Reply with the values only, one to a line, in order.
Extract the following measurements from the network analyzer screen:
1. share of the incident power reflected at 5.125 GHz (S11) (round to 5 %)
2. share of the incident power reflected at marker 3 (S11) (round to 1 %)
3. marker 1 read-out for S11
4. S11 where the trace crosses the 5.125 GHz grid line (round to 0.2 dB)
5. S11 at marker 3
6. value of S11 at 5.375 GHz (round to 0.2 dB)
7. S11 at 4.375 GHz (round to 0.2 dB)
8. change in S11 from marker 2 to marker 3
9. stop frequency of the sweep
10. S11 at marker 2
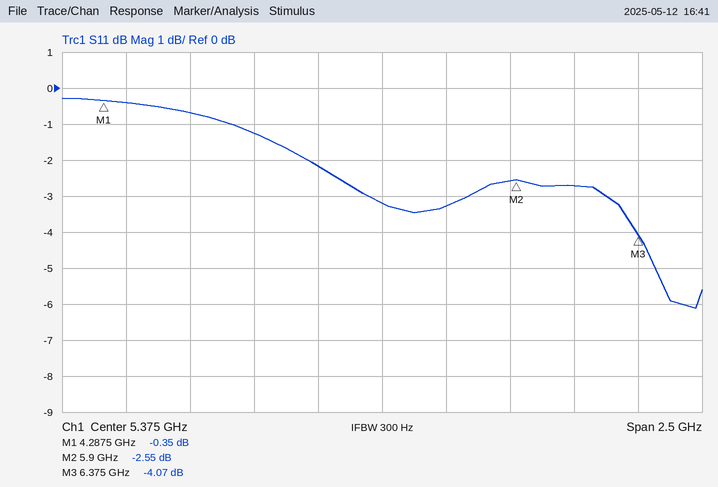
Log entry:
60 %
39 %
-0.35 dB
-2.2 dB
-4.07 dB
-3.2 dB
-0.4 dB
-1.52 dB
6.625 GHz
-2.55 dB
